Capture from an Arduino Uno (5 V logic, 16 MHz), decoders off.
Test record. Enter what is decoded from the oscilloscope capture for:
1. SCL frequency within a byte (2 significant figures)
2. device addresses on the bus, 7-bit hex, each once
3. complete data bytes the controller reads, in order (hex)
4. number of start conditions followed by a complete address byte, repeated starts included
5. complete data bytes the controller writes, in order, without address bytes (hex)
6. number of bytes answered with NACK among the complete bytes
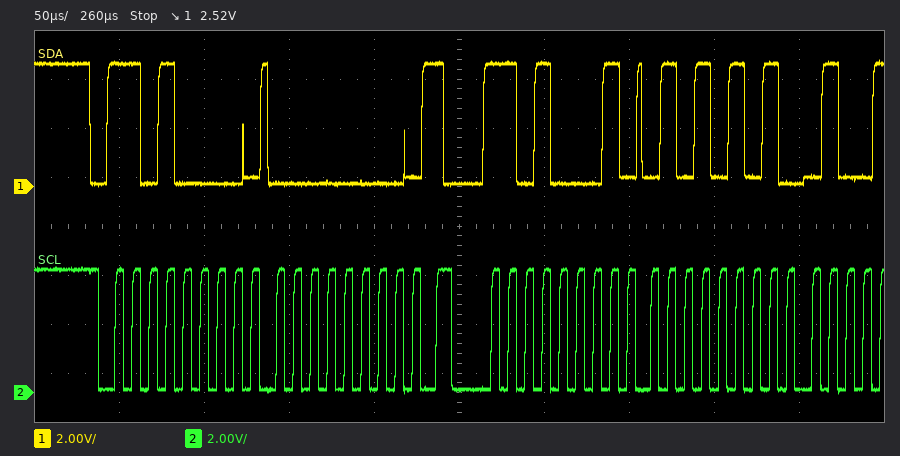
100 kHz
0x68
55
2
00
0
